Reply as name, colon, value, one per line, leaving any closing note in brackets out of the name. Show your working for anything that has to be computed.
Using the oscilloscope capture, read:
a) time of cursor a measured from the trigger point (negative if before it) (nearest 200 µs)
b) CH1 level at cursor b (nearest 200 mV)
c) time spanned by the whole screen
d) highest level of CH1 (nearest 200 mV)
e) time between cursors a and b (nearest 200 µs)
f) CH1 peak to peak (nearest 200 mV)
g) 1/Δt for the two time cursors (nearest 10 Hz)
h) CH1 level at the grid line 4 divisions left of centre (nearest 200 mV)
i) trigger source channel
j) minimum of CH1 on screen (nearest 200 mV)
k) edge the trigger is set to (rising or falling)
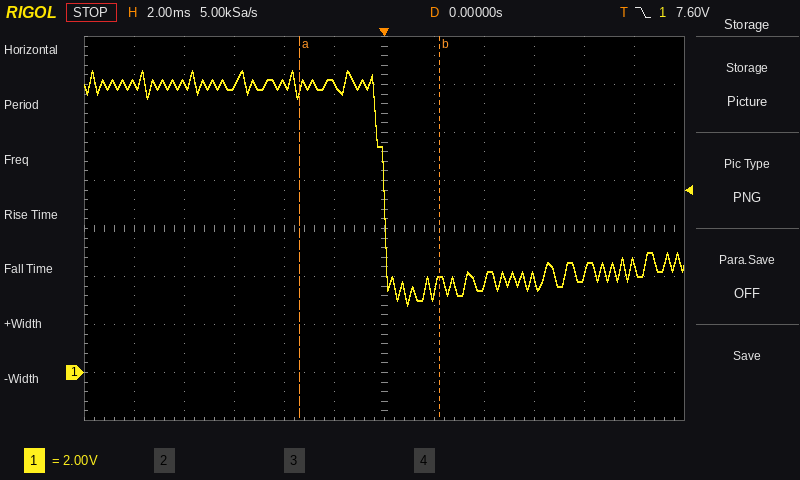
time of cursor a measured from the trigger point (negative if before it): -3.4 ms
CH1 level at cursor b: 3.8 V
time spanned by the whole screen: 24 ms
highest level of CH1: 12.6 V
time between cursors a and b: 5.6 ms
CH1 peak to peak: 12.6 V − (2.8 V) = 9.8 V
1/Δt for the two time cursors: 1 / 5.6 ms ≈ 180 Hz
CH1 level at the grid line 4 divisions left of centre: 12.0 V
trigger source channel: CH1
minimum of CH1 on screen: 2.8 V
edge the trigger is set to: falling
